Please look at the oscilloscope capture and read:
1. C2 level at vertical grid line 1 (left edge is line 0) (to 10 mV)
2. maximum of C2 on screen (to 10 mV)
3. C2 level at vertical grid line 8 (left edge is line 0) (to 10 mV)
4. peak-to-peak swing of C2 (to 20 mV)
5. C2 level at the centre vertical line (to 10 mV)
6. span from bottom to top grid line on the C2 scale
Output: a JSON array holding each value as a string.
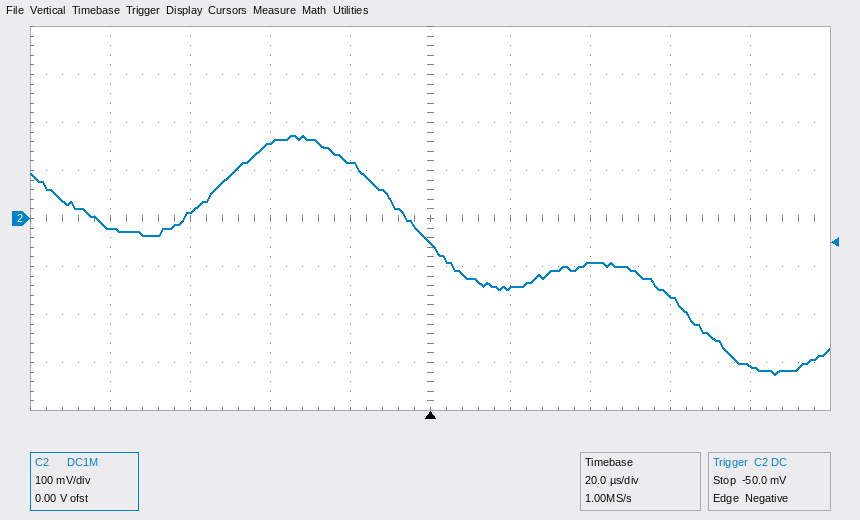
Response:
["-20 mV", "170 mV", "-160 mV", "500 mV", "-50 mV", "800 mV"]
